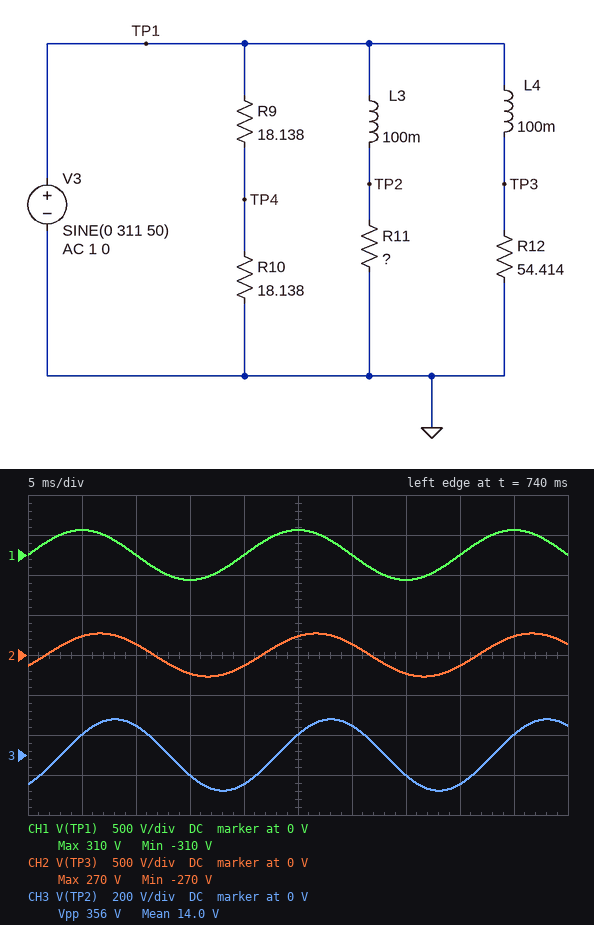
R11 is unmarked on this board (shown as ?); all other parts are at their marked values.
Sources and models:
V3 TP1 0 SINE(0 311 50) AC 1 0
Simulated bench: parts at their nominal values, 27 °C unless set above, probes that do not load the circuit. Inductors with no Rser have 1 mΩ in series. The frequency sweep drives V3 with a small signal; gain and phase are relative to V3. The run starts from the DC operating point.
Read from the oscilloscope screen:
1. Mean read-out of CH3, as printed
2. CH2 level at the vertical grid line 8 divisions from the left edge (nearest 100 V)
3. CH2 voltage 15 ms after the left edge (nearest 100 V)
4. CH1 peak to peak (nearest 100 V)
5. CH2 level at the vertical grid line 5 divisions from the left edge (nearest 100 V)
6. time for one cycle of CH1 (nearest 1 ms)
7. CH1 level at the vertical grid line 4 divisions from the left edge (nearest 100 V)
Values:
14.0 V
-100 V
-200 V
600 V
200 V
20 ms
0 V
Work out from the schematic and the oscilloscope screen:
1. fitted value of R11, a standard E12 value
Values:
22 Ω
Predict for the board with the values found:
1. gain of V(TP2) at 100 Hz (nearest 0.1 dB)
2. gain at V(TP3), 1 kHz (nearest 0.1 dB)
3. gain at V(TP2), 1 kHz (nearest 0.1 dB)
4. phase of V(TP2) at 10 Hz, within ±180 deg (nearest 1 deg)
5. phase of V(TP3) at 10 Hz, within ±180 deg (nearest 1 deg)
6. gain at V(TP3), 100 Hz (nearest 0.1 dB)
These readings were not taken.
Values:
-9.6 dB
-21.3 dB
-29.1 dB
-16 deg
-7 deg
-3.7 dB
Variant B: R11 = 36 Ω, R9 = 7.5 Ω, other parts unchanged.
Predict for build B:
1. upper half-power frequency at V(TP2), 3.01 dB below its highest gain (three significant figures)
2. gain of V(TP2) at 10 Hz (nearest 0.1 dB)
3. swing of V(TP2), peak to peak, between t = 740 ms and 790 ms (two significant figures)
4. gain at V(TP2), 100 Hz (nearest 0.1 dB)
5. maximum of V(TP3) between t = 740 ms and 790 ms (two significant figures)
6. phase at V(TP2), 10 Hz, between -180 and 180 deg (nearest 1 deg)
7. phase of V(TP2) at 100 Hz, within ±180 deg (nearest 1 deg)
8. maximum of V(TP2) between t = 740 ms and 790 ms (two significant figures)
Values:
57.3 Hz
-0.1 dB
470 V
-6.1 dB
270 V
-10 deg
-60 deg
230 V
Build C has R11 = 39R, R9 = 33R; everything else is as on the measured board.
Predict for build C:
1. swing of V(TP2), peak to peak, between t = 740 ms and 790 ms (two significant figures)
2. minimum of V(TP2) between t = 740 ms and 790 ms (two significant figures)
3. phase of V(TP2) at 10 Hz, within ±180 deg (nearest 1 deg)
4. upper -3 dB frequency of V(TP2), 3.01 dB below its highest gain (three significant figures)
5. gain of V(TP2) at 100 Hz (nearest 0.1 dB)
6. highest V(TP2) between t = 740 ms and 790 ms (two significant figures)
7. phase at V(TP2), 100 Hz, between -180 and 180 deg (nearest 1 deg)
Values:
480 V
-240 V
-9 deg
62.1 Hz
-5.6 dB
240 V
-58 deg
